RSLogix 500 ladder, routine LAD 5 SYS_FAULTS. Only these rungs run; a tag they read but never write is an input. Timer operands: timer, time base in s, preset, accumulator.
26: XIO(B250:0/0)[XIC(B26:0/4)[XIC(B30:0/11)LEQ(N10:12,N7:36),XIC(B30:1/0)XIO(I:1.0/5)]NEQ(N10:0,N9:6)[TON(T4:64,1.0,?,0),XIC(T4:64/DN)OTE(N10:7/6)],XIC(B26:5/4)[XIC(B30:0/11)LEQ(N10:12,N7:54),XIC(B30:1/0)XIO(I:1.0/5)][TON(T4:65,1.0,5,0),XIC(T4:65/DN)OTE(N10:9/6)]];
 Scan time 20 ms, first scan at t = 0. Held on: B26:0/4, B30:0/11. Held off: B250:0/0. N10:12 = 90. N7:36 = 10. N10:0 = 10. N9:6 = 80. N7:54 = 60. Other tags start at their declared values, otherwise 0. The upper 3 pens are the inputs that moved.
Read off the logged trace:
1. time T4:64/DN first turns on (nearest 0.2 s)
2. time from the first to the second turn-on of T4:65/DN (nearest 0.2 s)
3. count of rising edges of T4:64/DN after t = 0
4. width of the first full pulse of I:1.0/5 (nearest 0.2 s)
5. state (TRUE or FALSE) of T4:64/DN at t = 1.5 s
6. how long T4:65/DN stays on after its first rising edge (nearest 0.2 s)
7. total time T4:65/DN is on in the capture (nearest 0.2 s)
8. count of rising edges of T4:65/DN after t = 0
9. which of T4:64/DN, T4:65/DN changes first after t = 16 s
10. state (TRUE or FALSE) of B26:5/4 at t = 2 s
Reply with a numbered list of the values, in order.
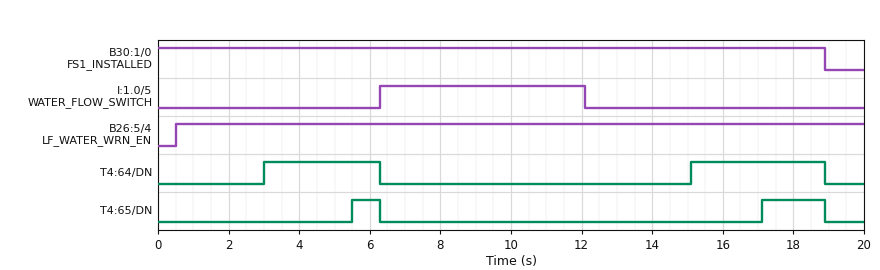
1. 3.0 s
2. 11.6 s
3. 2
4. 5.8 s
5. FALSE
6. 0.8 s
7. 2.6 s
8. 2
9. T4:65/DN
10. TRUE
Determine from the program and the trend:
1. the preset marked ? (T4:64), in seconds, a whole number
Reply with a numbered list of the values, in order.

1. 3 s
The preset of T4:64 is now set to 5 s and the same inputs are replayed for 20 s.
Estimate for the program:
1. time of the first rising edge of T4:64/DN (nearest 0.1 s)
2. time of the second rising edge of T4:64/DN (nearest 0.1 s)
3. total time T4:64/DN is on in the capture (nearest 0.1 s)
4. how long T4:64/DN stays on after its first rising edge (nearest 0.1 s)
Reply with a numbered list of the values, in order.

1. 5.0 s
2. 17.1 s
3. 3.1 s
4. 1.3 s
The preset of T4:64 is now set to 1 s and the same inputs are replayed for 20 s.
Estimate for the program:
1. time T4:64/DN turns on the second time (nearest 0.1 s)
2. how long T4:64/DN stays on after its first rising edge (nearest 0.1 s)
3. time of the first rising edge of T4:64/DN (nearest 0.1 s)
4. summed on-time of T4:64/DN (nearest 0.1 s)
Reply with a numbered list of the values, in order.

1. 13.1 s
2. 5.3 s
3. 1.0 s
4. 11.1 s
